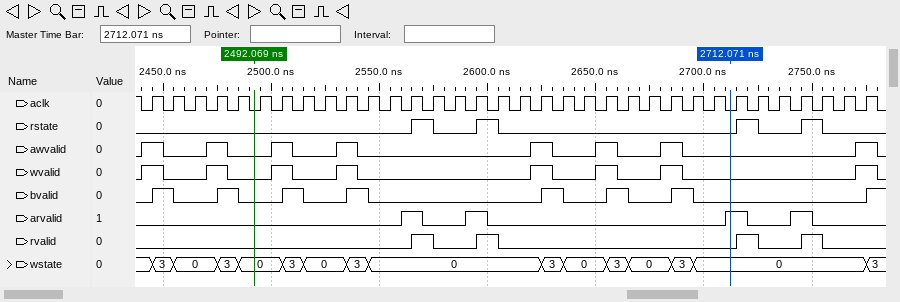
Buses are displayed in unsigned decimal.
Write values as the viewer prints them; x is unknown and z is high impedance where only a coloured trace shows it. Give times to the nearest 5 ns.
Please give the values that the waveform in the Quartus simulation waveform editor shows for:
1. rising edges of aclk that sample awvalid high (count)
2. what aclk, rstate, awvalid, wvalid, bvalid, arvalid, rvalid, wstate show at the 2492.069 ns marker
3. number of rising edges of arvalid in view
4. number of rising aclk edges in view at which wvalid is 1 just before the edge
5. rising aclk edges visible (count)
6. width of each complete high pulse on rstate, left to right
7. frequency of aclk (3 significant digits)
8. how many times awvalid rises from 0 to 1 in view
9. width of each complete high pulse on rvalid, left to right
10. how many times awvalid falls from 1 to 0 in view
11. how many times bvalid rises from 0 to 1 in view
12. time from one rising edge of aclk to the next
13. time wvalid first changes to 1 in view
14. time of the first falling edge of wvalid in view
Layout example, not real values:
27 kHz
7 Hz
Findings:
8
aclk=0, rstate=0, awvalid=0, wvalid=0, bvalid=0, arvalid=0, rvalid=0, wstate=0
4
8
34
10 ns, 10 ns, 10 ns, 10 ns
100 MHz
8
10 ns, 10 ns, 10 ns, 10 ns
8
8
10 ns
2440 ns
2450 ns
